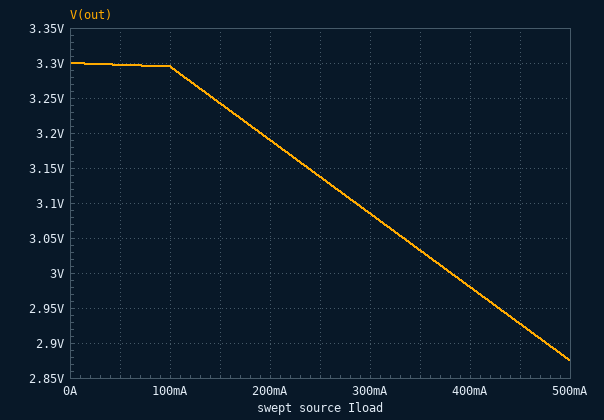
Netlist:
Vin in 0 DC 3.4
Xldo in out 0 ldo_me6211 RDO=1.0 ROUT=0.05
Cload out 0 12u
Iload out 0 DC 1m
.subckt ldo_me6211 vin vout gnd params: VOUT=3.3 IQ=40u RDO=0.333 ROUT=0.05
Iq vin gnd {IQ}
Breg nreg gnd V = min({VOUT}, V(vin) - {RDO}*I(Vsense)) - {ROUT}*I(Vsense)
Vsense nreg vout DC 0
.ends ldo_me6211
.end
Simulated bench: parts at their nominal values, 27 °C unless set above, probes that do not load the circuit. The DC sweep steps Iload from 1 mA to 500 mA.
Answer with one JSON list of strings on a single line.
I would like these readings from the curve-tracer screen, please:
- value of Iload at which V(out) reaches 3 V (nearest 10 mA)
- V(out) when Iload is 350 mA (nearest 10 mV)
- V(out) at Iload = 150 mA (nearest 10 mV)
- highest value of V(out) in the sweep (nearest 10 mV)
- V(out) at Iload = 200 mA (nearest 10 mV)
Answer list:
["380 mA", "3.03 V", "3.24 V", "3.30 V", "3.19 V"]
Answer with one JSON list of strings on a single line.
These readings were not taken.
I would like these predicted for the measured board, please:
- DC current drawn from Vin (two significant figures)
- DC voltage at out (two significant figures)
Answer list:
["40 µA", "3.3 V"]
